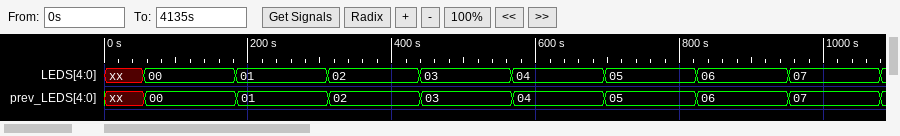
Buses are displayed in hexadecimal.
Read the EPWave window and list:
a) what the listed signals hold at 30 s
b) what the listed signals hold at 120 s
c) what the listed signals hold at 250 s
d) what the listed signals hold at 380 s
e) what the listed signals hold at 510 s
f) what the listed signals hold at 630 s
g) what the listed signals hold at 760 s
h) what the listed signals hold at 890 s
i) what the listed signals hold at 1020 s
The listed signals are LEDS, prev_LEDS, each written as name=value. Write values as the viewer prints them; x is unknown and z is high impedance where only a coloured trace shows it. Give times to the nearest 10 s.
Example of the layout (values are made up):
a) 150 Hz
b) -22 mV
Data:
a) LEDS=xx, prev_LEDS=xx
b) LEDS=00, prev_LEDS=00
c) LEDS=01, prev_LEDS=01
d) LEDS=02, prev_LEDS=02
e) LEDS=03, prev_LEDS=03
f) LEDS=04, prev_LEDS=04
g) LEDS=05, prev_LEDS=05
h) LEDS=06, prev_LEDS=06
i) LEDS=07, prev_LEDS=07
